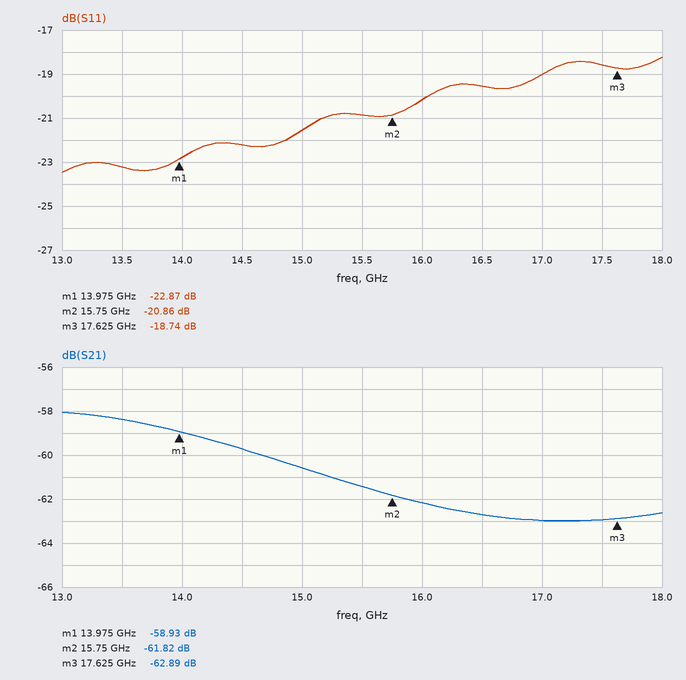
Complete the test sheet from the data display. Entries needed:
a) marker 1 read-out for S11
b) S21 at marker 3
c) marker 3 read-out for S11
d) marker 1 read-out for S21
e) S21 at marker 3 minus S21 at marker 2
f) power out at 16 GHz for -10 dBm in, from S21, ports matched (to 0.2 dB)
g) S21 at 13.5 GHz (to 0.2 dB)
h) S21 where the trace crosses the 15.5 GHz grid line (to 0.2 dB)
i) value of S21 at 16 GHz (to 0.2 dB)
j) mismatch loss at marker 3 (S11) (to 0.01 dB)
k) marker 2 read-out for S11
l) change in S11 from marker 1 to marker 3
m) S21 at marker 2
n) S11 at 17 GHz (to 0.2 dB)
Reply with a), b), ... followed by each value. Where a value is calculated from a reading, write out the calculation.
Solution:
a) -22.87 dB
b) -62.89 dB
c) -18.74 dB
d) -58.93 dB
e) -62.89 − (-61.82) = -1.07 dB
f) -10 dBm + (-62.2 dB) = -72.2 dBm
g) -58.4 dB
h) -61.4 dB
i) -62.2 dB
j) −10 log10(1 − 10^(-18.74/10)) ≈ 0.06 dB
k) -20.86 dB
l) -18.74 − (-22.87) = 4.13 dB
m) -61.82 dB
n) -19.0 dB
